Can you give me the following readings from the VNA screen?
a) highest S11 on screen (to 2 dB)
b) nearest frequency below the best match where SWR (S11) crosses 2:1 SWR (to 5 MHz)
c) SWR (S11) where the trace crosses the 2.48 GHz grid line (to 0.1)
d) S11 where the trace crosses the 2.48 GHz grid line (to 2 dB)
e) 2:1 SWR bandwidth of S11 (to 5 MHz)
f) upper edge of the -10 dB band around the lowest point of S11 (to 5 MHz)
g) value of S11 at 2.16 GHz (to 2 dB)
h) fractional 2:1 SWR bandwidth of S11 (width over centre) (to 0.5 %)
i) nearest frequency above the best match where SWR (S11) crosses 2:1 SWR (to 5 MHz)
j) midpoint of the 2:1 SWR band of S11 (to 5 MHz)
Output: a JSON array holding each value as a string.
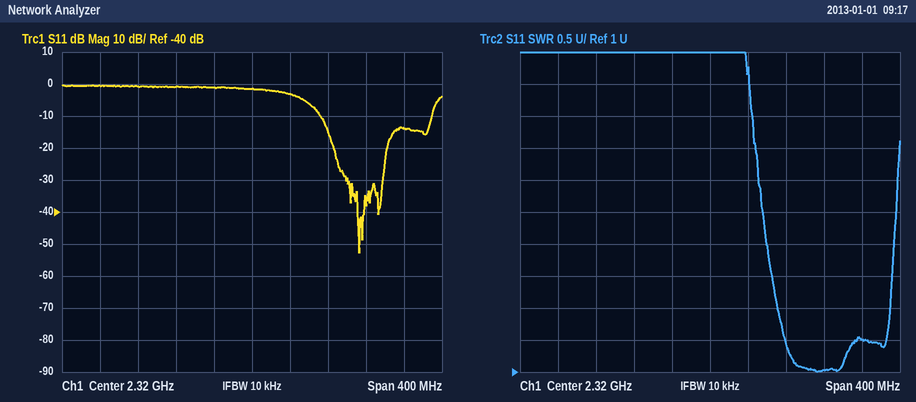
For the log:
["0 dB", "2.390 GHz", "1.5", "-14 dB", "120 MHz", "2.510 GHz", "0 dB", "5.0 %", "2.510 GHz", "2.450 GHz"]
